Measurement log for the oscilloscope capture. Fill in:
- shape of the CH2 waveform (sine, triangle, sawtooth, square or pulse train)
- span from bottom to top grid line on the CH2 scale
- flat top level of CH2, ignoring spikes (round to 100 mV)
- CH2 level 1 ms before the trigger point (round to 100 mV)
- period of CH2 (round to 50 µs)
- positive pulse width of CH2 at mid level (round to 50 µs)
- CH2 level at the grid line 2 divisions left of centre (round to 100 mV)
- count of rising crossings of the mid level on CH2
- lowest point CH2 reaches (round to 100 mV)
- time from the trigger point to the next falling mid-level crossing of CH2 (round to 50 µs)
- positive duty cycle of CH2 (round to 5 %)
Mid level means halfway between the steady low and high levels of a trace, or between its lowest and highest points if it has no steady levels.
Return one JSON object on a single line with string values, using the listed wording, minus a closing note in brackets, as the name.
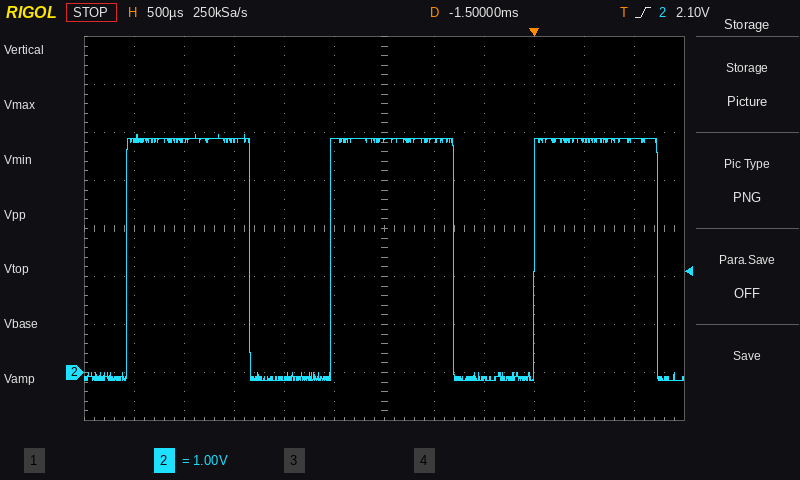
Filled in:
{"shape of the CH2 waveform": "pulse train", "span from bottom to top grid line on the CH2 scale": "8 V", "flat top level of CH2, ignoring spikes": "4.9 V", "CH2 level 1 ms before the trigger point": "4.8 V", "period of CH2": "2.05 ms", "positive pulse width of CH2 at mid level": "1.25 ms", "CH2 level at the grid line 2 divisions left of centre": "-100 mV", "count of rising crossings of the mid level on CH2": "3", "lowest point CH2 reaches": "-200 mV", "time from the trigger point to the next falling mid-level crossing of CH2": "1.25 ms", "positive duty cycle of CH2": "60 %"}
